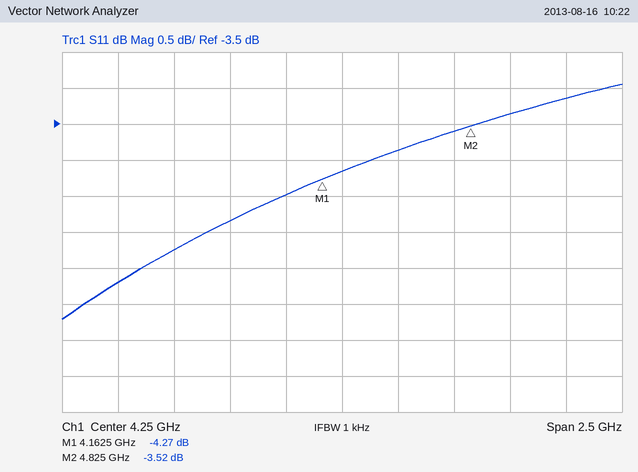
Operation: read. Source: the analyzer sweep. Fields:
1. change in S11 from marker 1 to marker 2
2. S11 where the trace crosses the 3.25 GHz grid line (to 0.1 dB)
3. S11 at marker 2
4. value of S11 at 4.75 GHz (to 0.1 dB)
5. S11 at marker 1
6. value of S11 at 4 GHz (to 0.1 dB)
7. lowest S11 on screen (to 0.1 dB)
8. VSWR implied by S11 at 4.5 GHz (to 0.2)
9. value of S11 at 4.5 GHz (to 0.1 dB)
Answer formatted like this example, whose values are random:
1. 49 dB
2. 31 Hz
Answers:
1. 0.75 dB
2. -5.7 dB
3. -3.52 dB
4. -3.6 dB
5. -4.27 dB
6. -4.5 dB
7. -6.2 dB
8. 4.6
9. -3.9 dB
